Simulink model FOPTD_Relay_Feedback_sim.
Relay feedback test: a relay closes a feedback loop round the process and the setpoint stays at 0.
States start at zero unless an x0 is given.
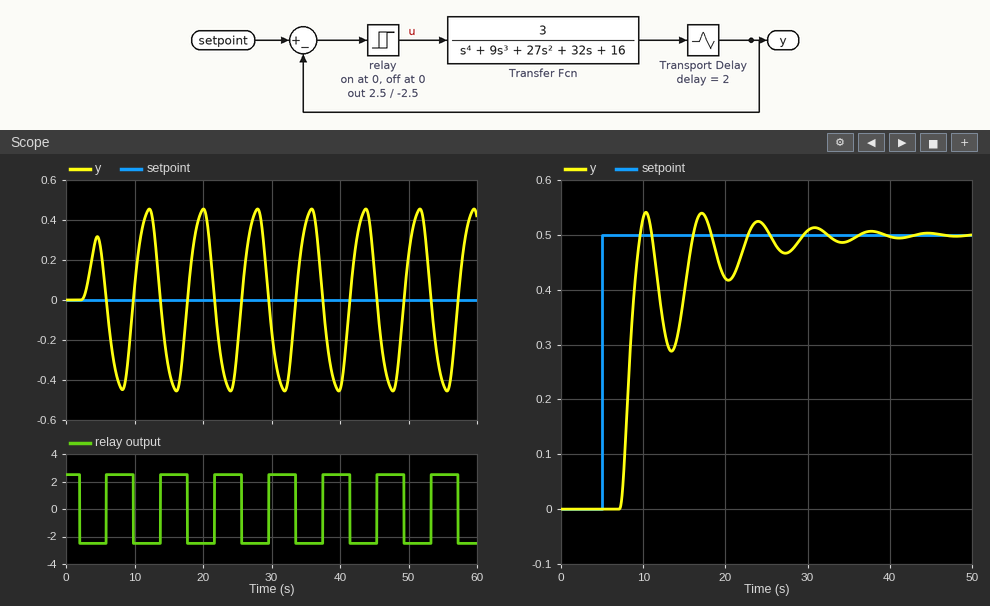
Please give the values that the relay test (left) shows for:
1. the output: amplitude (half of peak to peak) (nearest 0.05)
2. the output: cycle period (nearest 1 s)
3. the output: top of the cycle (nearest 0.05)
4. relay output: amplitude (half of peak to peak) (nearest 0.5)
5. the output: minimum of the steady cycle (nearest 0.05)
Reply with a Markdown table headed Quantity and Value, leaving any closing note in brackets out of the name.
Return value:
| Quantity | Value |
|---|---|
| the output: amplitude (half of peak to peak) | 0.45 |
| the output: cycle period | 8 s |
| the output: top of the cycle | 0.45 |
| relay output: amplitude (half of peak to peak) | 2.5 |
| the output: minimum of the steady cycle | -0.45 |
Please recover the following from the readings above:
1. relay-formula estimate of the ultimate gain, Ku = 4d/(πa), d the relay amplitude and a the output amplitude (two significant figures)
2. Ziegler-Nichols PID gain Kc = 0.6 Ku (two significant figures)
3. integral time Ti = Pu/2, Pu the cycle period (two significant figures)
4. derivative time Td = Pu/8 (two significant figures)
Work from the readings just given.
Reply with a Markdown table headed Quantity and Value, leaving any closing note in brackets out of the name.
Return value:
| Quantity | Value |
|---|---|
| relay-formula estimate of the ultimate gain, Ku = 4d/(πa), d the relay amplitude and a the output amplitude | 7.1 |
| Ziegler-Nichols PID gain Kc = 0.6 Ku | 4.3 |
| integral time Ti = Pu/2, Pu the cycle period | 4.0 s |
| derivative time Td = Pu/8 | 1.0 s |
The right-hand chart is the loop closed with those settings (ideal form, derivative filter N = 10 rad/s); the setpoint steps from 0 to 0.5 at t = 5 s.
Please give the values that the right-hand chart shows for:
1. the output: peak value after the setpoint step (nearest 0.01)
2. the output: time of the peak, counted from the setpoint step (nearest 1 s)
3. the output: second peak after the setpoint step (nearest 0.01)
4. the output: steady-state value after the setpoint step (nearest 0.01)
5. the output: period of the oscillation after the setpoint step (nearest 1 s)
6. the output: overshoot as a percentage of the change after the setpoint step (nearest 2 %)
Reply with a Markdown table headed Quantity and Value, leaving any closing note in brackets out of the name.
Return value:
| Quantity | Value |
|---|---|
| the output: peak value after the setpoint step | 0.54 |
| the output: time of the peak, counted from the setpoint step | 5 s |
| the output: second peak after the setpoint step | 0.54 |
| the output: steady-state value after the setpoint step | 0.50 |
| the output: period of the oscillation after the setpoint step | 7 s |
| the output: overshoot as a percentage of the change after the setpoint step | 8 % |
